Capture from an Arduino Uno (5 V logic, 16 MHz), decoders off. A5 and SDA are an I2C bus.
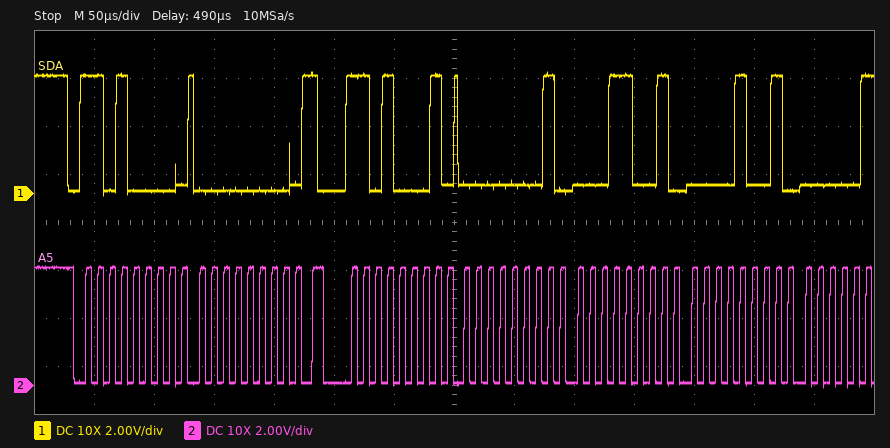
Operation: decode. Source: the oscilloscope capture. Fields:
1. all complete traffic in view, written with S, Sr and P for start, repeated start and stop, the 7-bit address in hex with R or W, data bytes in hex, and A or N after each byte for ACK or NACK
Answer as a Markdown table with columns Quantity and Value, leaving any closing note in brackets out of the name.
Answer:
| Quantity | Value |
|---|---|
| all complete traffic in view, written with S, Sr and P for start, repeated start and stop, the 7-bit address in hex with R or W, data bytes in hex, and A or N after each byte for ACK or NACK | S 68W A 00 A Sr 68R A 01 A 19 A 09 A |
